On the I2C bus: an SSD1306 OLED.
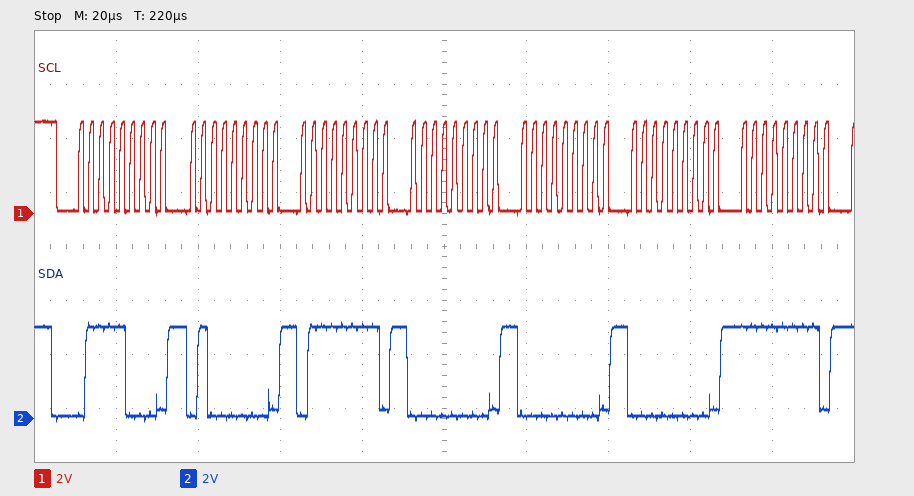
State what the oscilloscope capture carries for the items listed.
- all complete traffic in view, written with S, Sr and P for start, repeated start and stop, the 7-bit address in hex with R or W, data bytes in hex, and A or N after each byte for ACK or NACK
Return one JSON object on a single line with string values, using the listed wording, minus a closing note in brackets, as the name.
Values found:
{"all complete traffic in view, written with S, Sr and P for start, repeated start and stop, the 7-bit address in hex with R or W, data bytes in hex, and A or N after each byte for ACK or NACK": "S 3CW A 40 A 7F A 00 A 00 A 00 A FF A"}
